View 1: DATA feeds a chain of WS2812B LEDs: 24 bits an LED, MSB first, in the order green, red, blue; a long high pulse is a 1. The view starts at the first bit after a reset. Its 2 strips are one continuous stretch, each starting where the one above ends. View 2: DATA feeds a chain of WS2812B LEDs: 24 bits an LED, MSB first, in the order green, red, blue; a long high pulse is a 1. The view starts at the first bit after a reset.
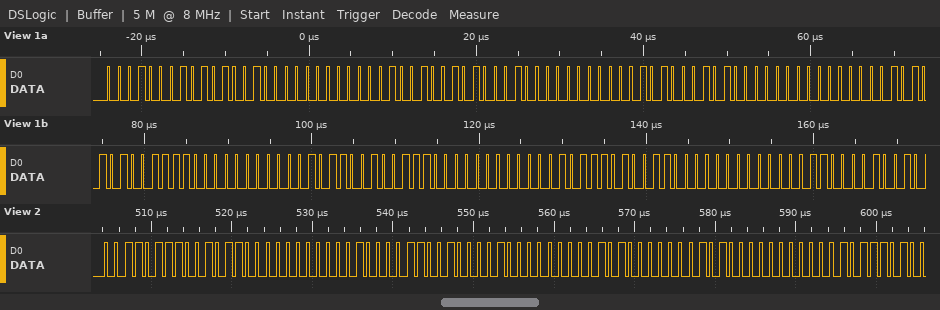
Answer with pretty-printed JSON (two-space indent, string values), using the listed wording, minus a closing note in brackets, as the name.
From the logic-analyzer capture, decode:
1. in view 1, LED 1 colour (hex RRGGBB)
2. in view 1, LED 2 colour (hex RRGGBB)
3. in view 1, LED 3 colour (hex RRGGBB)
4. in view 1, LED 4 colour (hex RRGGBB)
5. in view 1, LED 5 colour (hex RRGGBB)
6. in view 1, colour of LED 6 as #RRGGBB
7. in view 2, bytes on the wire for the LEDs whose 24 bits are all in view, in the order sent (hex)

{
  "in view 1, LED 1 colour": "#521100",
  "in view 1, LED 2 colour": "#511200",
  "in view 1, LED 3 colour": "#501400",
  "in view 1, LED 4 colour": "#4F1500",
  "in view 1, LED 5 colour": "#4E1600",
  "in view 1, colour of LED 6 as #RRGGBB": "#4C1700",
  "in view 2, bytes on the wire for the LEDs whose 24 bits are all in view, in the order sent": "37 2C 00 43 21 00 50 14 00"
}
